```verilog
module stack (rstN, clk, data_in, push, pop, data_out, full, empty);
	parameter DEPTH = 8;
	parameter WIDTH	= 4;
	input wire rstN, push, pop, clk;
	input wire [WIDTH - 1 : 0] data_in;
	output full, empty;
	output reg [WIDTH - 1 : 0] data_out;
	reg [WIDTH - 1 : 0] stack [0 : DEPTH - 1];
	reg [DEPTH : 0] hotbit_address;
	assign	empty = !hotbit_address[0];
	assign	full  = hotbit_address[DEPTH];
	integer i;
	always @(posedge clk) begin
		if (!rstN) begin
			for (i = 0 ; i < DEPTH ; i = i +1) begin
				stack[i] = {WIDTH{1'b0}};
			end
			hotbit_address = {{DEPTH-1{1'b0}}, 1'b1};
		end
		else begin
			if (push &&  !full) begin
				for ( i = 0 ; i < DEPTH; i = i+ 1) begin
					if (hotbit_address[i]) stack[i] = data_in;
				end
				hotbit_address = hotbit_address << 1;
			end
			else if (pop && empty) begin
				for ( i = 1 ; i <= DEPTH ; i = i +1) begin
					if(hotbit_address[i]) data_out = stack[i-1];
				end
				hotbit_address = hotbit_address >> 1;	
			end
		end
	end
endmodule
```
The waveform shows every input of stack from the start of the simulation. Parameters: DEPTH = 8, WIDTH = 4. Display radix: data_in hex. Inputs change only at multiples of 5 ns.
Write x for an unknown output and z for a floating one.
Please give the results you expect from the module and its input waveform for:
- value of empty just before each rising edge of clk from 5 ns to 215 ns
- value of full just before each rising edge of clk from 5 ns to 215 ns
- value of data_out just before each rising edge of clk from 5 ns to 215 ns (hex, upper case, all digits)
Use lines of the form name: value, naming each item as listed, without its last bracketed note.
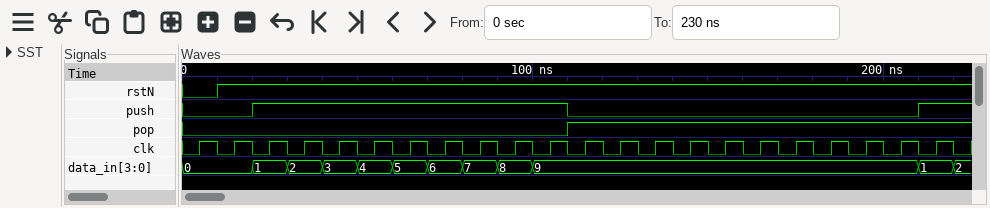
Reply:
value of empty just before each rising edge of clk from 5 ns to 215 ns: x 0 0 1 1 1 1 1 1 1 1 1 1 1 1 1 1 1 1 0 0 0
value of full just before each rising edge of clk from 5 ns to 215 ns: x 0 0 0 0 0 0 0 0 0 1 1 0 0 0 0 0 0 0 0 0 0
value of data_out just before each rising edge of clk from 5 ns to 215 ns: x, x, x, x, x, x, x, x, x, x, x, x, 8, 7, 6, 5, 4, 3, 2, 1, 1, 1
